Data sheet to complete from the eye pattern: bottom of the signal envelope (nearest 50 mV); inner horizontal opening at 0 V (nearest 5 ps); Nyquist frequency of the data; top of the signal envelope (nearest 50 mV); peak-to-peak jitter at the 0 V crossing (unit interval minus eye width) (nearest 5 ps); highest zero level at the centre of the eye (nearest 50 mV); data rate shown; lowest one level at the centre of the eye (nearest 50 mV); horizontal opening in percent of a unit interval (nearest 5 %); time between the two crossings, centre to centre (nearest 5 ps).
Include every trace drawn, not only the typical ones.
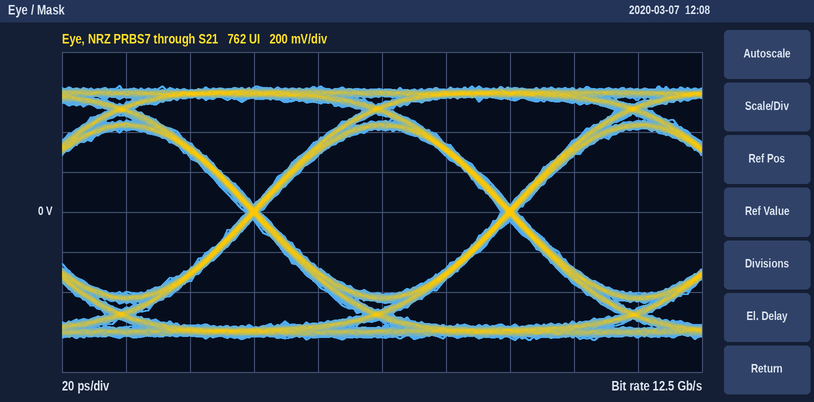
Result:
-650 mV
75 ps
6.25 GHz
650 mV
5 ps
-400 mV
12.5 Gb/s
400 mV
95 %
80 ps
